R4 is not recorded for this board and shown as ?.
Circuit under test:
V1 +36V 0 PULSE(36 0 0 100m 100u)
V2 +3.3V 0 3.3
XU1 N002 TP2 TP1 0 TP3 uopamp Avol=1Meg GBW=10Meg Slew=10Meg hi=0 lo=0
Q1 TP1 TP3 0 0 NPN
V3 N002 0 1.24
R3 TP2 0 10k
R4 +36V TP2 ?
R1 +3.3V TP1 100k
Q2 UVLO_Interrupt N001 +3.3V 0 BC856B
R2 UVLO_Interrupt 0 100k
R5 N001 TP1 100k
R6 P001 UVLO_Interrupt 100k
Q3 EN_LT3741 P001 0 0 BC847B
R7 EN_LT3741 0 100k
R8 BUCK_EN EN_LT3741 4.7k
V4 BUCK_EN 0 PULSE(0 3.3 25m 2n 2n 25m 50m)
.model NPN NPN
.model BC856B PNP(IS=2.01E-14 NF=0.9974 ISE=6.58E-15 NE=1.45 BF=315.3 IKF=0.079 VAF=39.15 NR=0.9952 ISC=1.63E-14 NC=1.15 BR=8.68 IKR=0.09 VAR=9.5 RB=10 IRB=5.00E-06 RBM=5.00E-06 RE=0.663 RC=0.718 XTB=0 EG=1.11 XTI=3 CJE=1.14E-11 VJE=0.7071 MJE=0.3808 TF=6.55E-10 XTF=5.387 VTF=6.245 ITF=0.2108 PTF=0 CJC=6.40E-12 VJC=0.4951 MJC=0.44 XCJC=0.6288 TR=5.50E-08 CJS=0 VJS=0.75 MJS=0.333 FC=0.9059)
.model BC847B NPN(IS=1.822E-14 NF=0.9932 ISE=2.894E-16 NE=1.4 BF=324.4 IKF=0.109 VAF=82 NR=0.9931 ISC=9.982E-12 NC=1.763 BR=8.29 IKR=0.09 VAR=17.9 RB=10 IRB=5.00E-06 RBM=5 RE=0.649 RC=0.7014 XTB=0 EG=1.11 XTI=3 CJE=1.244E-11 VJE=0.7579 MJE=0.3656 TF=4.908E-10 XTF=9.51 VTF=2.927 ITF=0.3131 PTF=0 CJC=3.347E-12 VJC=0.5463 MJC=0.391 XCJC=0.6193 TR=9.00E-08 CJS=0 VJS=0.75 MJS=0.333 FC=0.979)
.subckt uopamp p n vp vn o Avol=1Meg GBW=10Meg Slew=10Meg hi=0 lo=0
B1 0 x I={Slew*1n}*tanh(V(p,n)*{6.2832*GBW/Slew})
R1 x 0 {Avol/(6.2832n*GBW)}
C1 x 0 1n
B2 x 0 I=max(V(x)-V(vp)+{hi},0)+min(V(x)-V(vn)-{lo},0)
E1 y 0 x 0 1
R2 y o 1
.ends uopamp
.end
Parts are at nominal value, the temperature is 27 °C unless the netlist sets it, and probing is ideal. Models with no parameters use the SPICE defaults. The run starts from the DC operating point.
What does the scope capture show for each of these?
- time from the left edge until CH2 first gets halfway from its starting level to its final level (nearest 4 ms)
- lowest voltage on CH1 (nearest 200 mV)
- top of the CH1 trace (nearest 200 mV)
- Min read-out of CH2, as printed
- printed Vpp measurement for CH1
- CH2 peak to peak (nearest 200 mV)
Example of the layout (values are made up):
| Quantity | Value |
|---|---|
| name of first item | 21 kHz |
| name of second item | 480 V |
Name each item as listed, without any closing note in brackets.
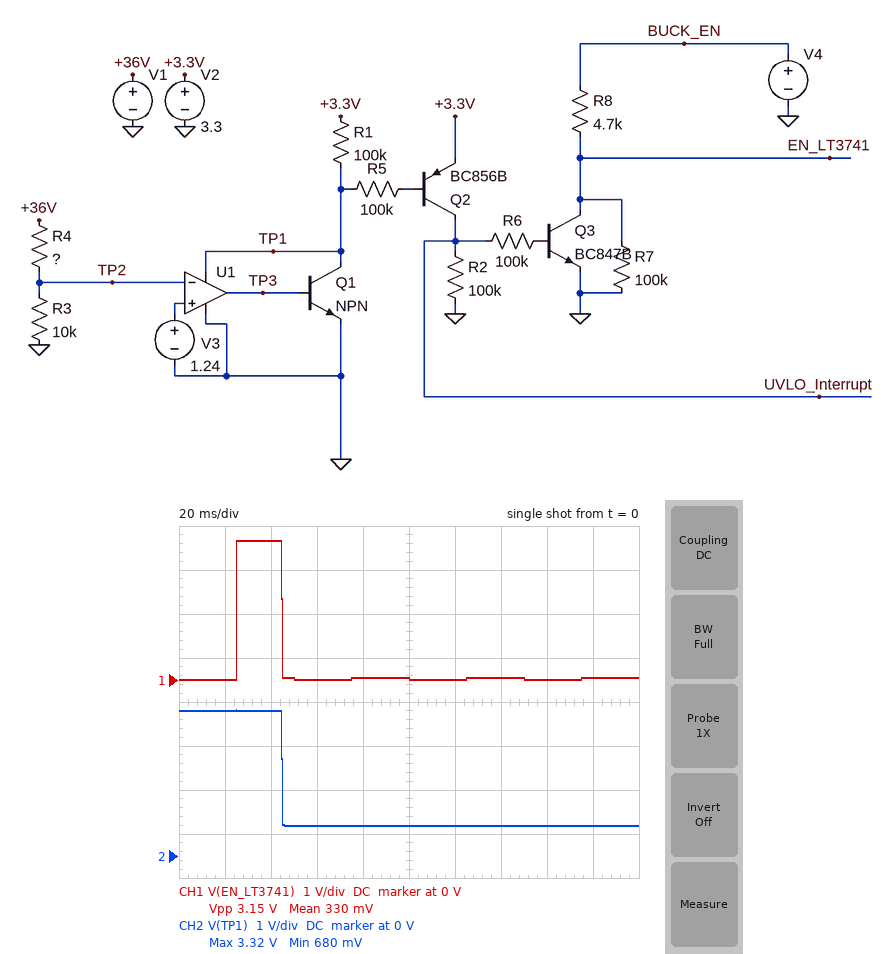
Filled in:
| Quantity | Value |
|---|---|
| time from the left edge until CH2 first gets halfway from its starting level to its final level | 44 ms |
| lowest voltage on CH1 | 0 V |
| top of the CH1 trace | 3.2 V |
| Min read-out of CH2, as printed | 680 mV |
| printed Vpp measurement for CH1 | 3.15 V |
| CH2 peak to peak | 2.6 V |
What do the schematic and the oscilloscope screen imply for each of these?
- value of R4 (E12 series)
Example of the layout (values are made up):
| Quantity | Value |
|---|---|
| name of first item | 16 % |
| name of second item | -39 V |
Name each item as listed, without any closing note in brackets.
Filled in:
| Quantity | Value |
|---|---|
| value of R4 | 150 kΩ |
